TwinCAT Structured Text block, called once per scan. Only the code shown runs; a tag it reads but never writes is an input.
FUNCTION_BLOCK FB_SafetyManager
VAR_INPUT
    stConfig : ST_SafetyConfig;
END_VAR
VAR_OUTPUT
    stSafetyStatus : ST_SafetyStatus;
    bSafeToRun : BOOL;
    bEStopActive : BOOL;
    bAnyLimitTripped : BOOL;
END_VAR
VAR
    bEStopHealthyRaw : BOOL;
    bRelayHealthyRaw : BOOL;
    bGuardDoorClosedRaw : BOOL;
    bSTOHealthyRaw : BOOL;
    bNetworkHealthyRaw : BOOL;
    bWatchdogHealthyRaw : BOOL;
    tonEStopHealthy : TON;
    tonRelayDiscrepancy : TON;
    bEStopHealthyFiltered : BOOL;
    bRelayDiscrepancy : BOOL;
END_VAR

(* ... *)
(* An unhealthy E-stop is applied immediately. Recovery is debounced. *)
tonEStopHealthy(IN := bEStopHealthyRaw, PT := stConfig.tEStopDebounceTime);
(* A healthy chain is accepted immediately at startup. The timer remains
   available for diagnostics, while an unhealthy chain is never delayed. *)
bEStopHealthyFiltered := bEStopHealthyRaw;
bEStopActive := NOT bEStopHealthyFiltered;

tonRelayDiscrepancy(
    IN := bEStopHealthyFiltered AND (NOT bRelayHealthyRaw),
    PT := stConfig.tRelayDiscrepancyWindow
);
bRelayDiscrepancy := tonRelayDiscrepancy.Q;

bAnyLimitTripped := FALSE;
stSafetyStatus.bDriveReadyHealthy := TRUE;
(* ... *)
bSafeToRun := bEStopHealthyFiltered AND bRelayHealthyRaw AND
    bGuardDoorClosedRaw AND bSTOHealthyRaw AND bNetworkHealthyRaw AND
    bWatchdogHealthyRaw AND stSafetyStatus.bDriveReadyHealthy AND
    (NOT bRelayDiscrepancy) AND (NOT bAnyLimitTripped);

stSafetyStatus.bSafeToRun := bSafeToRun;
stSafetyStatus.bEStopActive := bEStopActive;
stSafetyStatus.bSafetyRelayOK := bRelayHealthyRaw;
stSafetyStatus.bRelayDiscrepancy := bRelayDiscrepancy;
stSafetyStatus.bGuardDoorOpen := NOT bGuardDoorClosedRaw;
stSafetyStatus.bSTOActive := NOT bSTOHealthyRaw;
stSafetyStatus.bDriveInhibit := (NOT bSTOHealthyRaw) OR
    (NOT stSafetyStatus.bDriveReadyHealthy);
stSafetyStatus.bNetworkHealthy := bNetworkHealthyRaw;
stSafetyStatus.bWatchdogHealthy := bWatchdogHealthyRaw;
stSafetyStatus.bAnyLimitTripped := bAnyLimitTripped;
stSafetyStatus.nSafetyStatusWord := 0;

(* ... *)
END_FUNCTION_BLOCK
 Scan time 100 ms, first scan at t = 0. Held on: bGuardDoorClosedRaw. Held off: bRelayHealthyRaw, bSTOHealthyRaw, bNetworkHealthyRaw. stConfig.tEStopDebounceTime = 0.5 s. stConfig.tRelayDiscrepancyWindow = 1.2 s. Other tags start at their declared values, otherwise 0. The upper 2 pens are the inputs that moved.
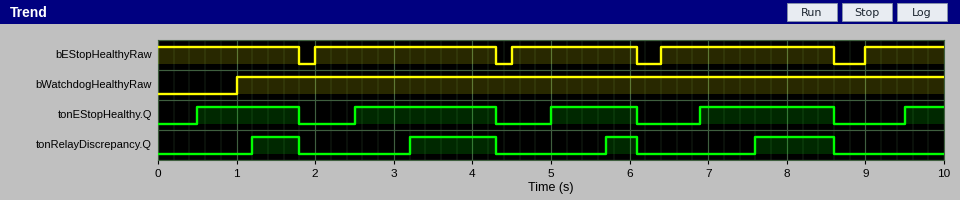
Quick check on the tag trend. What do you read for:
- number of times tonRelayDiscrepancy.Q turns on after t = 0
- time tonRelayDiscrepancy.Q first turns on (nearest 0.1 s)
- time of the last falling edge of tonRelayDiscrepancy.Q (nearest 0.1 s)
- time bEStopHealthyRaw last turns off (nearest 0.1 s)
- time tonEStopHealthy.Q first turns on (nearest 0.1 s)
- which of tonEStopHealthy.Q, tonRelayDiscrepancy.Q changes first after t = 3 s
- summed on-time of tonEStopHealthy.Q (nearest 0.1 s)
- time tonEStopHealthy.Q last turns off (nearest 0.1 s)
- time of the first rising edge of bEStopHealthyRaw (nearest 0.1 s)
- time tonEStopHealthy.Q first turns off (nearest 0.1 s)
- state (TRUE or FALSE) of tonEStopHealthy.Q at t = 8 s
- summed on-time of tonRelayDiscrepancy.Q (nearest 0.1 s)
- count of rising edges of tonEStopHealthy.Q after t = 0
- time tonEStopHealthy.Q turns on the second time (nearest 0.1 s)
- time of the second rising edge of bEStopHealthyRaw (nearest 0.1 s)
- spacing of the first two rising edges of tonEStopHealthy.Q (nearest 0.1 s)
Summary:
4
1.2 s
8.6 s
8.6 s
0.5 s
tonRelayDiscrepancy.Q
6.4 s
8.6 s
2.0 s
1.8 s
TRUE
3.1 s
5
2.5 s
4.5 s
2.0 s
